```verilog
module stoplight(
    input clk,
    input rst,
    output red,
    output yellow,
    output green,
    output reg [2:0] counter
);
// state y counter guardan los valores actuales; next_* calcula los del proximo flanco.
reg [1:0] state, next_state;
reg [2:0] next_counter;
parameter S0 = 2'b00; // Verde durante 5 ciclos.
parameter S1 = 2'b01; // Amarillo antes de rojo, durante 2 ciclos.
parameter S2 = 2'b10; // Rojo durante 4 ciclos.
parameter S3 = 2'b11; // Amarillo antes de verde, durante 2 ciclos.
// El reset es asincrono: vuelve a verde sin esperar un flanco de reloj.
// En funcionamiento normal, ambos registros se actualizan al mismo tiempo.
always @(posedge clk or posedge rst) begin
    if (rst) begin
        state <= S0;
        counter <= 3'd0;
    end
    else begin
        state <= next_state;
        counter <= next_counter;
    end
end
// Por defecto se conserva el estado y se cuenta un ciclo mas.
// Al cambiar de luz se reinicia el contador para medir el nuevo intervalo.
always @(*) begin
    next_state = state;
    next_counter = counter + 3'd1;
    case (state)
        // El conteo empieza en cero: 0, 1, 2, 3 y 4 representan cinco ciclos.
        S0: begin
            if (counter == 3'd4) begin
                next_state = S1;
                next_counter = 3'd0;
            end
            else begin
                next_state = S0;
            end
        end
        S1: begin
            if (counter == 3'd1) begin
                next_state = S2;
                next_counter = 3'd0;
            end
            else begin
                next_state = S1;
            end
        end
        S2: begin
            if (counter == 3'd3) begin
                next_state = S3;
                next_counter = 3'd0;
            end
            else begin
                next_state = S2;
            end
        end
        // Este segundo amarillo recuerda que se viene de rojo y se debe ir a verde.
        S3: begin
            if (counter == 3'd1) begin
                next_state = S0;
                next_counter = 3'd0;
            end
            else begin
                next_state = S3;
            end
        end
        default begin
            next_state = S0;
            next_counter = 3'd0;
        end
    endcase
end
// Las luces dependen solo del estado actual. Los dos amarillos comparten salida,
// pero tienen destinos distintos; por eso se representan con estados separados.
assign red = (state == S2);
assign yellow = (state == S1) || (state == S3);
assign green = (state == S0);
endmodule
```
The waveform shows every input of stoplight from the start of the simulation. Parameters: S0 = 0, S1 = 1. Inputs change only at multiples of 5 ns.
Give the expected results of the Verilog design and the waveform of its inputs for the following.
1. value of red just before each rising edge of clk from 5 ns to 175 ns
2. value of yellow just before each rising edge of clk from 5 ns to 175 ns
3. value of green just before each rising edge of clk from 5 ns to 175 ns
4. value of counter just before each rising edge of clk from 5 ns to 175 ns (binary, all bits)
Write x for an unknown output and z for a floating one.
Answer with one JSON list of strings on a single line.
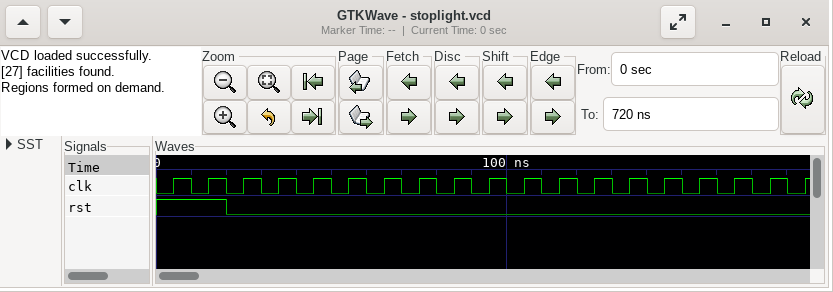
["0 0 0 0 0 0 0 0 0 1 1 1 1 0 0 0 0 0", "0 0 0 0 0 0 0 1 1 0 0 0 0 1 1 0 0 0", "1 1 1 1 1 1 1 0 0 0 0 0 0 0 0 1 1 1", "000, 000, 000, 001, 010, 011, 100, 000, 001, 000, 001, 010, 011, 000, 001, 000, 001, 010"]
